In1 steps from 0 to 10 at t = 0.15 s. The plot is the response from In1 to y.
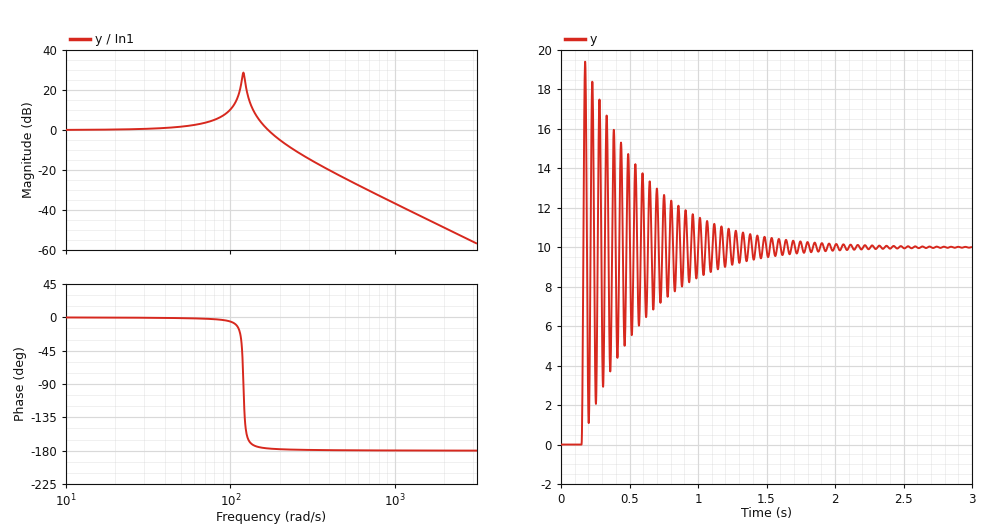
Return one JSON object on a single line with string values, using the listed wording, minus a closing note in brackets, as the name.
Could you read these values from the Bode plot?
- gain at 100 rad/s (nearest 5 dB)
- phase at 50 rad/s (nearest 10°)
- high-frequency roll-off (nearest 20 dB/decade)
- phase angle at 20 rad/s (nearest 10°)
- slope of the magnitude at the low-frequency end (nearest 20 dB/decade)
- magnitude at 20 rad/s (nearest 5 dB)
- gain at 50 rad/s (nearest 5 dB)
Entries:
{"gain at 100 rad/s": "10 dB", "phase at 50 rad/s": "0°", "high-frequency roll-off": "-40 dB/decade", "phase angle at 20 rad/s": "0°", "slope of the magnitude at the low-frequency end": "0 dB/decade", "magnitude at 20 rad/s": "0 dB", "gain at 50 rad/s": "0 dB"}
